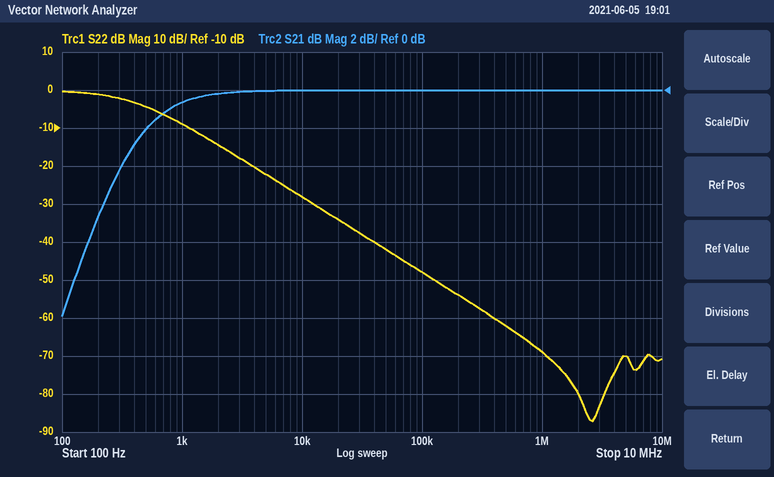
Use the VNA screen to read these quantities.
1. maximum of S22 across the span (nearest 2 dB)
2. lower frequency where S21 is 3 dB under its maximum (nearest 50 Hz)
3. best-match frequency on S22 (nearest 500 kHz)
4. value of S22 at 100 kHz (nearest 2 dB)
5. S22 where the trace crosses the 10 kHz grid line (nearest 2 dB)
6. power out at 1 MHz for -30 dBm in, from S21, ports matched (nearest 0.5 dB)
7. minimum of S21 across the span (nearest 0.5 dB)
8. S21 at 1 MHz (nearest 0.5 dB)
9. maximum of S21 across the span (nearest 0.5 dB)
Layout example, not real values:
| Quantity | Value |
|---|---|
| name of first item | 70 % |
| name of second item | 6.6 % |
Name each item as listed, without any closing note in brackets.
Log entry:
| Quantity | Value |
|---|---|
| maximum of S22 across the span | 0 dB |
| lower frequency where S21 is 3 dB under its maximum | 400 Hz |
| best-match frequency on S22 | 2.5 MHz |
| value of S22 at 100 kHz | -48 dB |
| S22 where the trace crosses the 10 kHz grid line | -28 dB |
| power out at 1 MHz for -30 dBm in, from S21, ports matched | -30.0 dBm |
| minimum of S21 across the span | -12.0 dB |
| S21 at 1 MHz | 0.0 dB |
| maximum of S21 across the span | 0.0 dB |
